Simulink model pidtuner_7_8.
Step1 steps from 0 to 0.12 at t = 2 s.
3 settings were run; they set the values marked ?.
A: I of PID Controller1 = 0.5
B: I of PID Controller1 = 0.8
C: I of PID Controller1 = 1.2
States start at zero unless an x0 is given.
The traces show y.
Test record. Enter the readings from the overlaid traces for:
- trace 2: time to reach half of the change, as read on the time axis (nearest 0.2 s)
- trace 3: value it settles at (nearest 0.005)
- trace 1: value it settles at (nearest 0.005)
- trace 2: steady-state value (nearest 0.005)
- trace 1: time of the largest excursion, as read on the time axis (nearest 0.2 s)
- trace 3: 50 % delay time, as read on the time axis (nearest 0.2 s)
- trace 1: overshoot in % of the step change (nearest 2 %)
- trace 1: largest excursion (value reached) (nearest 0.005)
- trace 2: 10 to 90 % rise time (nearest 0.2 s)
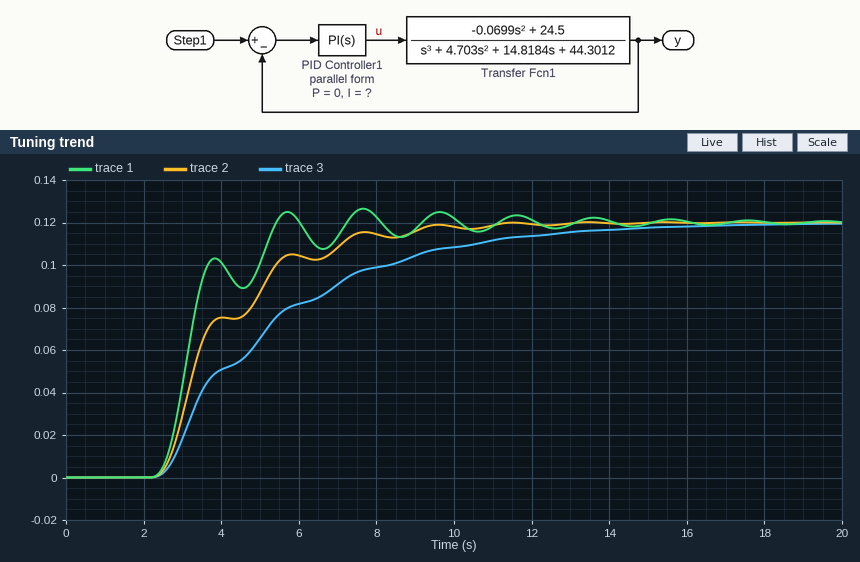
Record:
3.4 s
0.120
0.120
0.120
7.6 s
4.8 s
6 %
0.125
4.2 s
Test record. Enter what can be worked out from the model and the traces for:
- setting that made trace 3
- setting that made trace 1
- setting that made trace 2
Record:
A
C
B
